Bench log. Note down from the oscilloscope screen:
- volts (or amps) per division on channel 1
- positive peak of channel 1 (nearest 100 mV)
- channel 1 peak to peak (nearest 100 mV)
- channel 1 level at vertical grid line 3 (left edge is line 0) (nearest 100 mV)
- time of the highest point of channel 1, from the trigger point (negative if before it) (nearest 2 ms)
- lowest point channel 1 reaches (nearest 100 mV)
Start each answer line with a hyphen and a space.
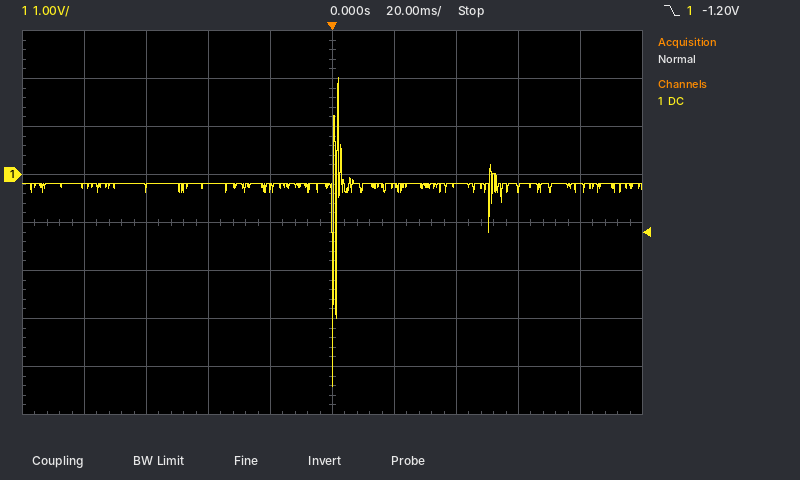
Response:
- 1 V
- 2.0 V
- 6.4 V
- -200 mV
- +2 ms
- -4.4 V
